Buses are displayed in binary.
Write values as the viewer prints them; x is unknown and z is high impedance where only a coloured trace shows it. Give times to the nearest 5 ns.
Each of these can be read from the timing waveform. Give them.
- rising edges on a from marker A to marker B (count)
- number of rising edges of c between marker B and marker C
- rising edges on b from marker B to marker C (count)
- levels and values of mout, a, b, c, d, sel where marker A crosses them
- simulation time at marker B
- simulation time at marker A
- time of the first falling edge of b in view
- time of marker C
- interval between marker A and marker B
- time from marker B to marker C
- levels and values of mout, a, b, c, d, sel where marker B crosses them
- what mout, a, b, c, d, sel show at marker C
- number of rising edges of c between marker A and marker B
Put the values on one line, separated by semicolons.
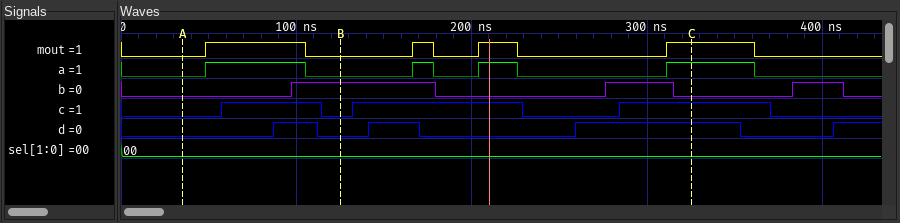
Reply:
1; 2; 1; mout=0, a=0, b=0, c=0, d=0, sel=00; 125 ns; 35 ns; 180 ns; 325 ns; 90 ns; 200 ns; mout=0, a=0, b=1, c=0, d=0, sel=00; mout=1, a=1, b=0, c=1, d=1, sel=00; 1
